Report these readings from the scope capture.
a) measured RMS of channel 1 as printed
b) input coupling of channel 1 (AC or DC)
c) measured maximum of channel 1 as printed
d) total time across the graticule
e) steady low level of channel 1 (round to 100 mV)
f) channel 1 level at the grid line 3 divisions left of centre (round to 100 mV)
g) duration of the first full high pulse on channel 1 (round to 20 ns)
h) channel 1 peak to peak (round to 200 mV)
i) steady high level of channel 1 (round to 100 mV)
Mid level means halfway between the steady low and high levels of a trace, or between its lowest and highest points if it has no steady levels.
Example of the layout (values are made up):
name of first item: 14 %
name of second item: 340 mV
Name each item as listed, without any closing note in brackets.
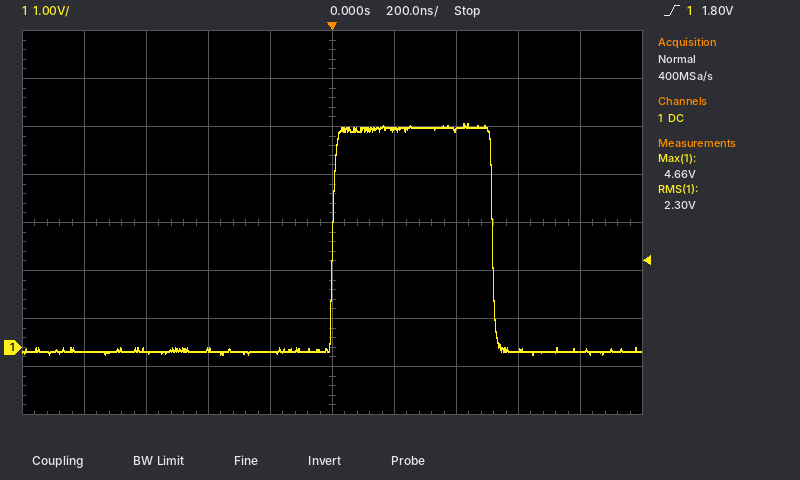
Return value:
measured RMS of channel 1 as printed: 2.30 V
input coupling of channel 1: DC
measured maximum of channel 1 as printed: 4.66 V
total time across the graticule: 2 µs
steady low level of channel 1: -100 mV
channel 1 level at the grid line 3 divisions left of centre: -100 mV
duration of the first full high pulse on channel 1: 520 ns
channel 1 peak to peak: 4.8 V
steady high level of channel 1: 4.6 V
